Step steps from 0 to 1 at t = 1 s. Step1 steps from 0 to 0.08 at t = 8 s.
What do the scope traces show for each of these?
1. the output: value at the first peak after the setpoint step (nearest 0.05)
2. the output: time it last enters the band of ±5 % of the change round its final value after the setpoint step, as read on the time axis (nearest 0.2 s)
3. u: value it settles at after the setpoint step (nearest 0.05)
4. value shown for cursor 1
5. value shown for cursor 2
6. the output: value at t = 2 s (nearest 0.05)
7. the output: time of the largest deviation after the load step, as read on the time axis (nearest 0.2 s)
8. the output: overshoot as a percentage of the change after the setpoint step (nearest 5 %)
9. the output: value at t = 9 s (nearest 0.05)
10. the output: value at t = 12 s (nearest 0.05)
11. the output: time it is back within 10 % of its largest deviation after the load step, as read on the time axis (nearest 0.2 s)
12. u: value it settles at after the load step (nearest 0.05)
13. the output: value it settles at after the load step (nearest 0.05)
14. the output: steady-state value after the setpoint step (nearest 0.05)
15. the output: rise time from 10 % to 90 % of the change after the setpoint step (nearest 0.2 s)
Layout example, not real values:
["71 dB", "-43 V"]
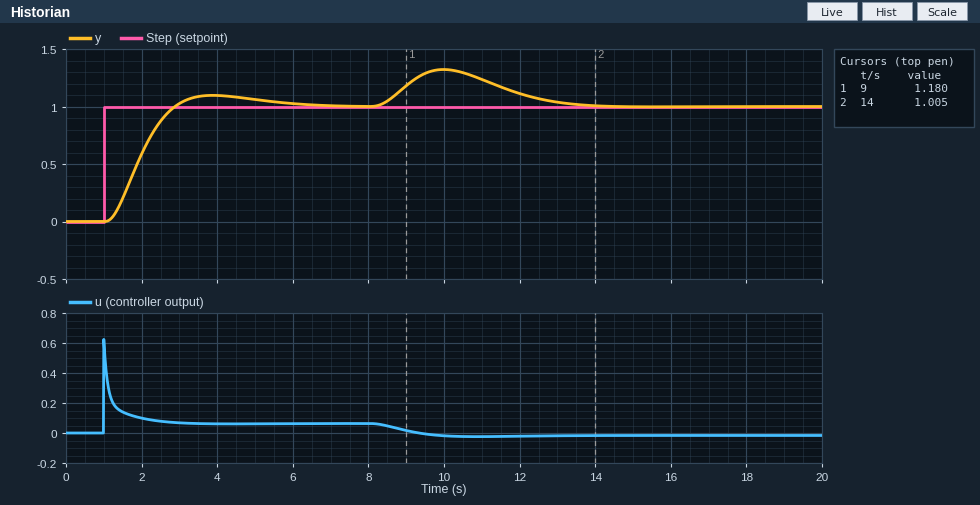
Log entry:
["1.10", "5.2 s", "0.05", "1.180", "1.005", "0.60", "10.0 s", "10 %", "1.20", "1.10", "13.2 s", "0.00", "1.00", "1.00", "1.2 s"]
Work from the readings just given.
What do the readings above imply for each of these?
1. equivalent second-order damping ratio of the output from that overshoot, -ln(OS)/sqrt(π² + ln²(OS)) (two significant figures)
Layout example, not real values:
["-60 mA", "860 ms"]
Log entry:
["0.59"]
